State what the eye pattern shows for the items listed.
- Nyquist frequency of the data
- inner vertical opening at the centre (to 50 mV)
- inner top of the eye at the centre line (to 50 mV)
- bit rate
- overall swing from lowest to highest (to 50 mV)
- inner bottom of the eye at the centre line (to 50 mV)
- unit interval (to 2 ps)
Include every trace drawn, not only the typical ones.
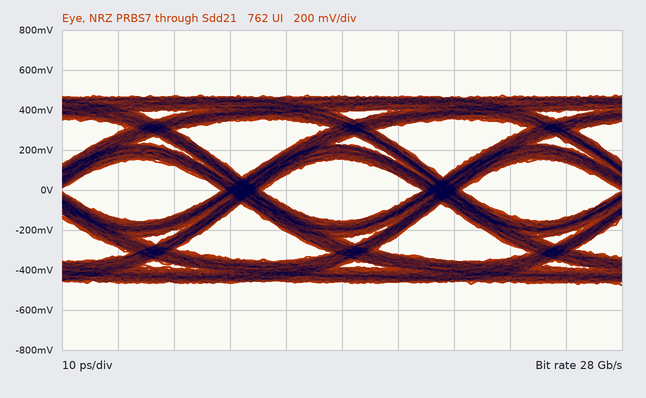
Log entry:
14 GHz
300 mV
150 mV
28 Gb/s
950 mV
-150 mV
36 ps
